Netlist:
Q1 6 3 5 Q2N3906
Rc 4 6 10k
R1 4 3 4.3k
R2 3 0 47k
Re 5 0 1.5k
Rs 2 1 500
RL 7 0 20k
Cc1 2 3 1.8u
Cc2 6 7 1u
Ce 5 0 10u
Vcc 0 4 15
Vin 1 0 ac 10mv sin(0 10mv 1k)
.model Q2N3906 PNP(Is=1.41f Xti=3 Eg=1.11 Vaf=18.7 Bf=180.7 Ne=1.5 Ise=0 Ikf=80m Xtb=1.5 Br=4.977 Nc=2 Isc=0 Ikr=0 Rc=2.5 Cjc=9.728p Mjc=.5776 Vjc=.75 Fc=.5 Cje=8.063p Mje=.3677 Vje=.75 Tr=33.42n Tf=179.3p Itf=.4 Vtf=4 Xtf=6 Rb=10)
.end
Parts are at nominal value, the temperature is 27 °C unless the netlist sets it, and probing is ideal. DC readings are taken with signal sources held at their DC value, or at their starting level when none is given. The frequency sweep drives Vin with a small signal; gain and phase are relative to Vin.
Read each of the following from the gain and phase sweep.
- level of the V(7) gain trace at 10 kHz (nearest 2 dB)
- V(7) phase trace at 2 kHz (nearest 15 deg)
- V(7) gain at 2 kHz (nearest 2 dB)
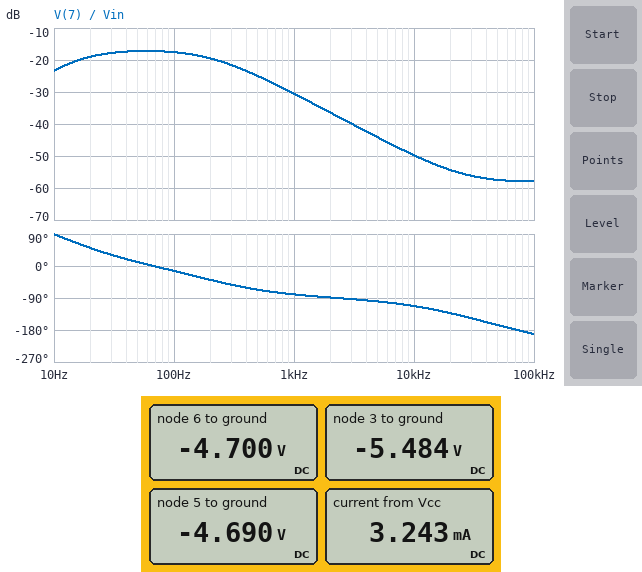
-50 dB
-90 deg
-36 dB
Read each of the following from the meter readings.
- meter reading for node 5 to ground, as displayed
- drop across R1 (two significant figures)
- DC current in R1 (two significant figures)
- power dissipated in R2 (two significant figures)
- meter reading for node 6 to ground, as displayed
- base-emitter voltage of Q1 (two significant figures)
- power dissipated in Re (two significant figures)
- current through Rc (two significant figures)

-4.690 V
9.5 V
2.2 mA
640 µW
-4.700 V
-790 mV
15 mW
1.0 mA
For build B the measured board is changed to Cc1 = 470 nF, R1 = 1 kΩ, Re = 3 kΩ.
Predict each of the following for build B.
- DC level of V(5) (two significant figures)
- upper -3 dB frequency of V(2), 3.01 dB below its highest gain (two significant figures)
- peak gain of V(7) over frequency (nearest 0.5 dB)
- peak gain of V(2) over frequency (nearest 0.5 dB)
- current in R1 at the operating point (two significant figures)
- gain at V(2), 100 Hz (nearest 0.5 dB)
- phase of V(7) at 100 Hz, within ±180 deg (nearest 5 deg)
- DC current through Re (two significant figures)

-11 V
680 Hz
-27.5 dB
0 dB
3.4 mA
0 dB
10 deg
3.6 mA
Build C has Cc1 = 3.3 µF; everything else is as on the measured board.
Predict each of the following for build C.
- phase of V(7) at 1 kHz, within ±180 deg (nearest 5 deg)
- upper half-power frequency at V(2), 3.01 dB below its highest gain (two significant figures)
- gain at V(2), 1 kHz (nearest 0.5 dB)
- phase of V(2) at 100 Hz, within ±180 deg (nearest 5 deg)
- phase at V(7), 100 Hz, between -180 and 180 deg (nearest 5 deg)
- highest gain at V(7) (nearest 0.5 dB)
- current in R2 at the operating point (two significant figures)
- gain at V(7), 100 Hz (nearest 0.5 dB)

-85 deg
120 Hz
-18.0 dB
-35 deg
-25 deg
-13.5 dB
120 µA
-14.5 dB
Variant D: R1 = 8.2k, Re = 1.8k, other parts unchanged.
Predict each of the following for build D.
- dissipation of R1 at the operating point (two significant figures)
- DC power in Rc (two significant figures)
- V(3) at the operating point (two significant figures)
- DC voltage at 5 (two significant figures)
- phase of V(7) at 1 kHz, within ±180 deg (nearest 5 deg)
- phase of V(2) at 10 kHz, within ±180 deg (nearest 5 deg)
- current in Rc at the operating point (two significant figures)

13 mW
12 mW
-4.8 V
-4.0 V
-90 deg
-20 deg
1.1 mA
